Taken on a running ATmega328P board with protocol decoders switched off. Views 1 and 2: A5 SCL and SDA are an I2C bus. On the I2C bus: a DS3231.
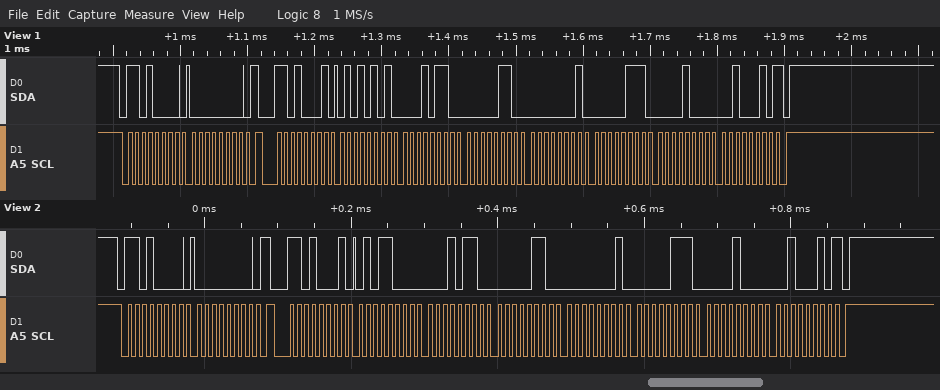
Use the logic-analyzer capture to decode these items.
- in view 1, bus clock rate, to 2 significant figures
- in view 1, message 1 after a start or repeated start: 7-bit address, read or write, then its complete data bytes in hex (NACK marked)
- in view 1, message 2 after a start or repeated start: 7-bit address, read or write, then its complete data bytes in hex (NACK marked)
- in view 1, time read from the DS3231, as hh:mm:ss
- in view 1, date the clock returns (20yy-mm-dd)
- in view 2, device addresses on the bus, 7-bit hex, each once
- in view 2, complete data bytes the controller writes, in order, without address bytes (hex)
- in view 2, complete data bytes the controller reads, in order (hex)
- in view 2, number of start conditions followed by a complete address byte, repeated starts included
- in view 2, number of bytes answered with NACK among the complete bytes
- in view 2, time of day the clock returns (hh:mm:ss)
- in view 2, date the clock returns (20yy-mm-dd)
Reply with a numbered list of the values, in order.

1. 100 kHz
2. 0x68 write: 00
3. 0x68 read: 55 16 06 01 07 08 22 NACK
4. 06:16:55
5. 2022-08-07
6. 0x68
7. 00
8. 58 16 06 01 07 08 22
9. 2
10. 1
11. 06:16:58
12. 2022-08-07
